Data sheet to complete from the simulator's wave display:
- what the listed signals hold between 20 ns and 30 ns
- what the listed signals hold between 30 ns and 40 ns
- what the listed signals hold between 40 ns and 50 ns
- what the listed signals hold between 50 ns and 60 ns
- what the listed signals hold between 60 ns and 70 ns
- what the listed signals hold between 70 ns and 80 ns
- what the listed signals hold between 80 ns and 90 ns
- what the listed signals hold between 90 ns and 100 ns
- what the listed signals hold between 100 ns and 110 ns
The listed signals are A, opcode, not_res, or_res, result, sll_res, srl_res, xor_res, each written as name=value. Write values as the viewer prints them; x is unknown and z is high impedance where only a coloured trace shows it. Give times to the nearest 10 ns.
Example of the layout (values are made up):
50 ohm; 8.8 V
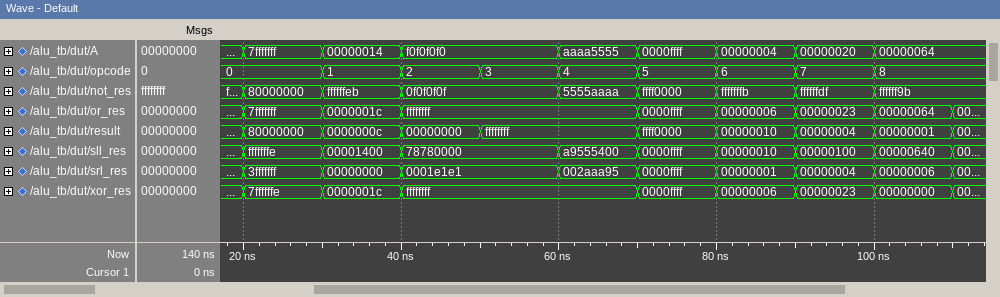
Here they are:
A=7fffffff, opcode=0, not_res=80000000, or_res=7fffffff, result=80000000, sll_res=fffffffe, srl_res=3fffffff, xor_res=7ffffffe; A=00000014, opcode=1, not_res=ffffffeb, or_res=0000001c, result=0000000c, sll_res=00001400, srl_res=00000000, xor_res=0000001c; A=f0f0f0f0, opcode=2, not_res=0f0f0f0f, or_res=ffffffff, result=00000000, sll_res=78780000, srl_res=0001e1e1, xor_res=ffffffff; A=f0f0f0f0, opcode=3, not_res=0f0f0f0f, or_res=ffffffff, result=ffffffff, sll_res=78780000, srl_res=0001e1e1, xor_res=ffffffff; A=aaaa5555, opcode=4, not_res=5555aaaa, or_res=ffffffff, result=ffffffff, sll_res=a9555400, srl_res=002aaa95, xor_res=ffffffff; A=0000ffff, opcode=5, not_res=ffff0000, or_res=0000ffff, result=ffff0000, sll_res=0000ffff, srl_res=0000ffff, xor_res=0000ffff; A=00000004, opcode=6, not_res=fffffffb, or_res=00000006, result=00000010, sll_res=00000010, srl_res=00000001, xor_res=00000006; A=00000020, opcode=7, not_res=ffffffdf, or_res=00000023, result=00000004, sll_res=00000100, srl_res=00000004, xor_res=00000023; A=00000064, opcode=8, not_res=ffffff9b, or_res=00000064, result=00000001, sll_res=00000640, srl_res=00000006, xor_res=00000000
